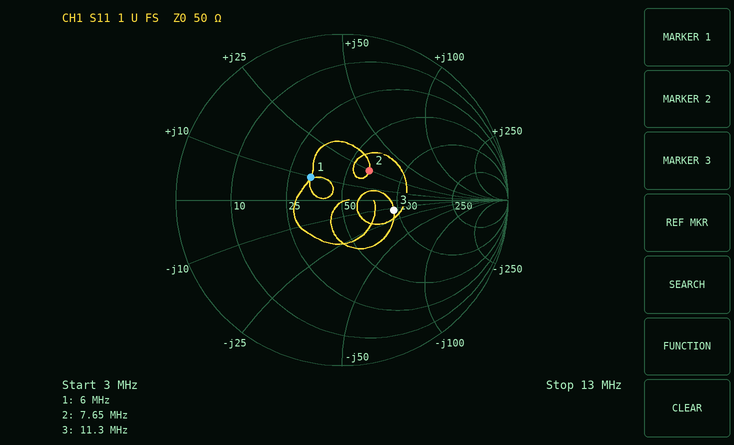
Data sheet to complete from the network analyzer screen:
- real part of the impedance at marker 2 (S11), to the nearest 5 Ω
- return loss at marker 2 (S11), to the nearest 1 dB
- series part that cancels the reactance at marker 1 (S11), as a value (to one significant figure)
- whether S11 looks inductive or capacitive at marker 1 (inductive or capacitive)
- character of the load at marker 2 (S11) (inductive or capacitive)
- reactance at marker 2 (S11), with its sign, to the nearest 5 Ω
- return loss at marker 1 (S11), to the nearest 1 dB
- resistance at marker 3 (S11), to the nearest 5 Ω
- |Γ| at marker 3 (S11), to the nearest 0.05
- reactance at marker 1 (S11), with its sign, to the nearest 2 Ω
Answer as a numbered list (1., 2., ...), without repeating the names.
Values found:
1. 65 Ω
2. 12 dB
3. 3 nF
4. inductive
5. inductive
6. +25 Ω
7. 13 dB
8. 95 Ω
9. 0.30
10. +10 Ω
